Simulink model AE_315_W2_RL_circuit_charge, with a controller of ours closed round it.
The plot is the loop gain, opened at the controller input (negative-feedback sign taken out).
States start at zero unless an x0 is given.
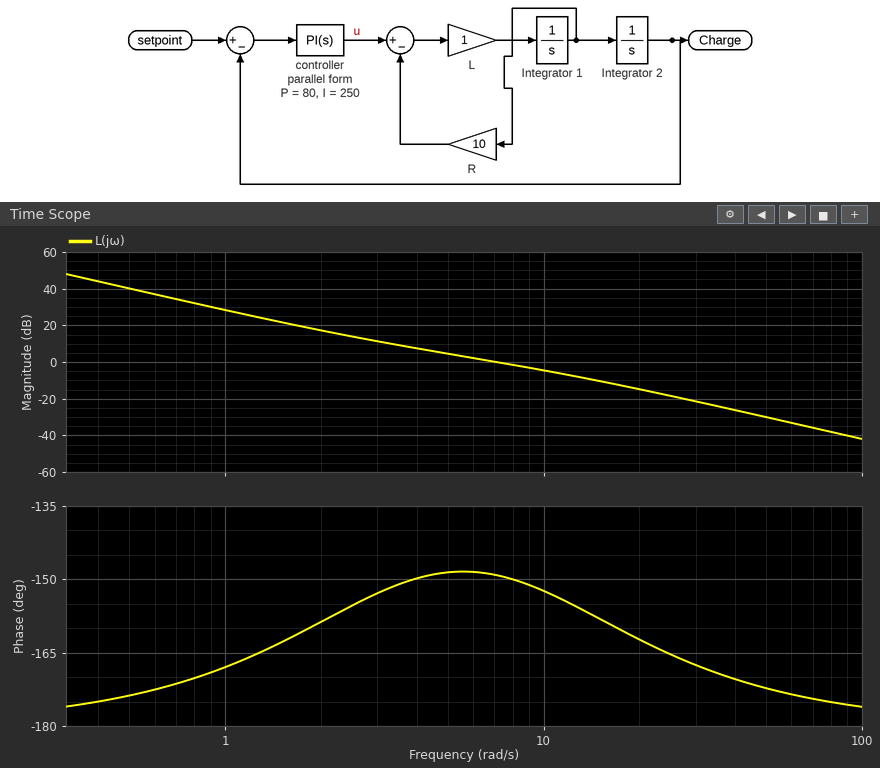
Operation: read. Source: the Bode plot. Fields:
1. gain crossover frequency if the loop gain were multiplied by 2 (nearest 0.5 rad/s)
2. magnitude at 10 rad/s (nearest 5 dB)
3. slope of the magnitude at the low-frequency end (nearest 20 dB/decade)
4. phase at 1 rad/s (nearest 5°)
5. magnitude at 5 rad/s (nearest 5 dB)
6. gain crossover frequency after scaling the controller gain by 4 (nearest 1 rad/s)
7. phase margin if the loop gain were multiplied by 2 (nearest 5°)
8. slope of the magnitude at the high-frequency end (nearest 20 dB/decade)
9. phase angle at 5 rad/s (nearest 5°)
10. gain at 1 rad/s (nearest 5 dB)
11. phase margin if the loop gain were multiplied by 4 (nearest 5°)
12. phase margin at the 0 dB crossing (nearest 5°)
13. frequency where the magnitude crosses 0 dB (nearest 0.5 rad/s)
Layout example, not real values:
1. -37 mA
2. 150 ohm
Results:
1. 11.0 rad/s
2. -5 dB
3. -40 dB/decade
4. -170°
5. 5 dB
6. 17 rad/s
7. 25°
8. -40 dB/decade
9. -150°
10. 30 dB
11. 20°
12. 30°
13. 7.0 rad/s
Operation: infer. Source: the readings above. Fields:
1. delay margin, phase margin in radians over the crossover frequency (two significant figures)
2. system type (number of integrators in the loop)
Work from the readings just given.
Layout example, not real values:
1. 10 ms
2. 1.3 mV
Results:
1. 0.075 s
2. 2
